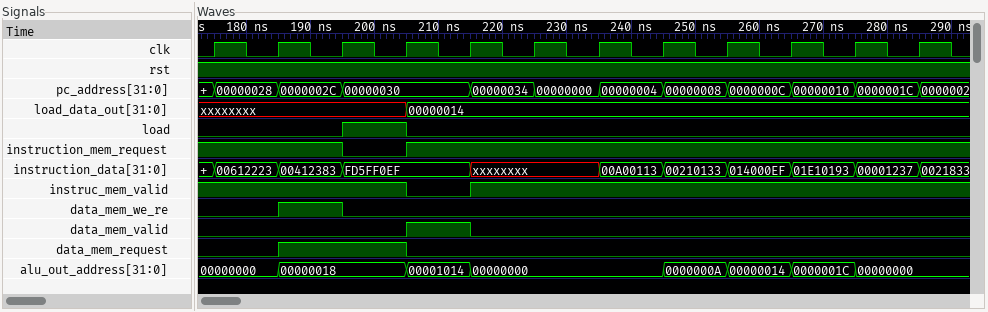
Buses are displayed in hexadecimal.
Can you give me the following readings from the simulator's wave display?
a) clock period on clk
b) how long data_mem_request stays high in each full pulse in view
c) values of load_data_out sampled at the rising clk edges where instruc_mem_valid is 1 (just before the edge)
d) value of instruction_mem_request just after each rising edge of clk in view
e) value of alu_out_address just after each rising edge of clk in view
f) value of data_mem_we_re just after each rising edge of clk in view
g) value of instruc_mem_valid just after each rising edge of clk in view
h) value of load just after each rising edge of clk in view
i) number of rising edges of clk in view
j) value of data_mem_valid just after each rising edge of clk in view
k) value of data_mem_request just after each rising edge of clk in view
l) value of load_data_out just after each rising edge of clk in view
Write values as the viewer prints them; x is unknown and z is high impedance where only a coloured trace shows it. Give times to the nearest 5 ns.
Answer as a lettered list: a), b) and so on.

a) 10 ns
b) 20 ns
c) xxxxxxxx, xxxxxxxx, xxxxxxxx, xxxxxxxx, 00000014, 00000014, 00000014, 00000014, 00000014, 00000014, 00000014
d) 1 1 0 1 1 1 1 1 1 1 1 1
e) 00000000, 00000018, 00000018, 00001014, 00000000, 00000000, 00000000, 0000000A, 00000014, 0000001C, 00000000, 00000000
f) 0 1 0 0 0 0 0 0 0 0 0 0
g) 1 1 1 0 1 1 1 1 1 1 1 1
h) 0 0 1 0 0 0 0 0 0 0 0 0
i) 12
j) 0 0 0 1 0 0 0 0 0 0 0 0
k) 0 1 1 0 0 0 0 0 0 0 0 0
l) xxxxxxxx, xxxxxxxx, xxxxxxxx, 00000014, 00000014, 00000014, 00000014, 00000014, 00000014, 00000014, 00000014, 00000014
